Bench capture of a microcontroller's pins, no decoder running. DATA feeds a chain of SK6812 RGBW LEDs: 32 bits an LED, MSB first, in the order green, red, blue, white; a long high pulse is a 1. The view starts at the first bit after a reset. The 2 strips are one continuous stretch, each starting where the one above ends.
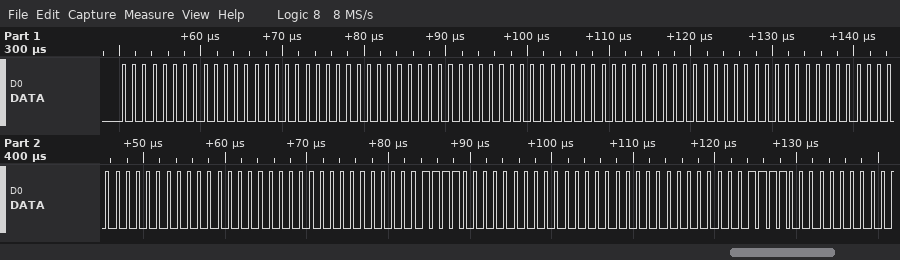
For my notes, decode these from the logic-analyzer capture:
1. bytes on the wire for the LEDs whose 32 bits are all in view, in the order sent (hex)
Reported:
00 00 00 00 00 00 00 00 00 00 00 00 00 1E 00 00
